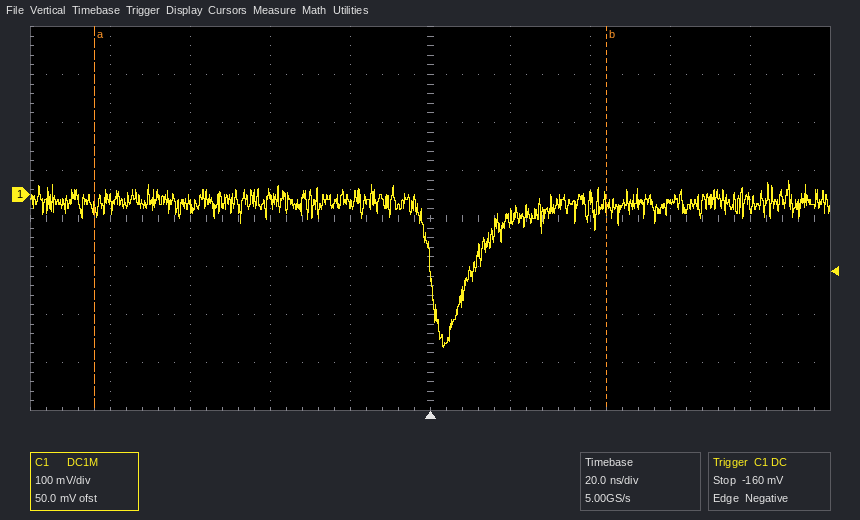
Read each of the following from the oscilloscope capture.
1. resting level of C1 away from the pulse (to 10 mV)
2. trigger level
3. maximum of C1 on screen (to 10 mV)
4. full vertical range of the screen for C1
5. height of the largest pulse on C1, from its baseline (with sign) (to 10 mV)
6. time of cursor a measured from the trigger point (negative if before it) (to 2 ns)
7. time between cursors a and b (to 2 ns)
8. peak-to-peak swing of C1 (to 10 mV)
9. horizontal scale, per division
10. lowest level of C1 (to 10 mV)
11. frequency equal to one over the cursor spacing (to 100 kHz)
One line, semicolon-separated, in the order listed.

-20 mV; -160 mV; 30 mV; 800 mV; -300 mV; -84 ns; 128 ns; 350 mV; 20 ns; -320 mV; 7.8 MHz
